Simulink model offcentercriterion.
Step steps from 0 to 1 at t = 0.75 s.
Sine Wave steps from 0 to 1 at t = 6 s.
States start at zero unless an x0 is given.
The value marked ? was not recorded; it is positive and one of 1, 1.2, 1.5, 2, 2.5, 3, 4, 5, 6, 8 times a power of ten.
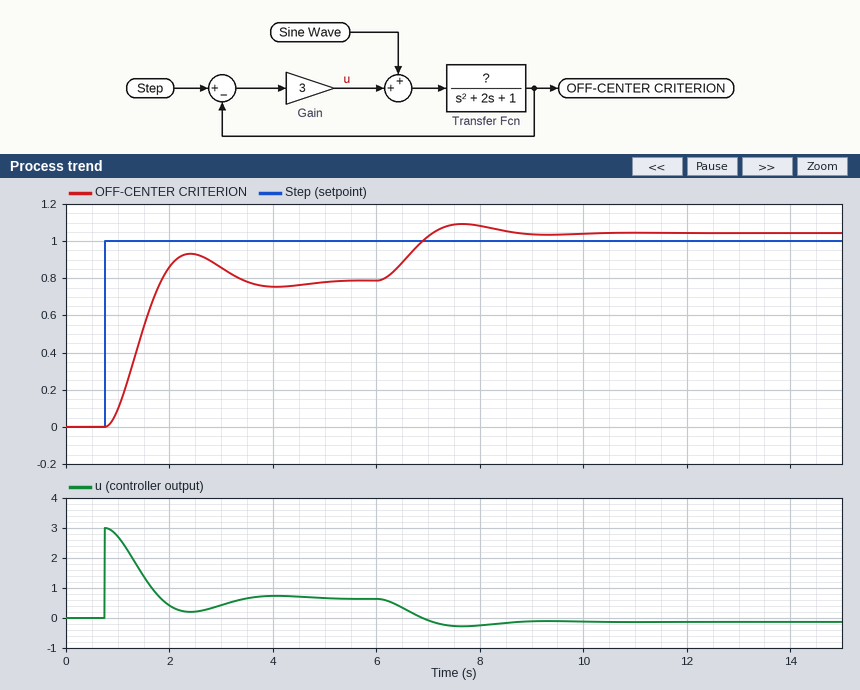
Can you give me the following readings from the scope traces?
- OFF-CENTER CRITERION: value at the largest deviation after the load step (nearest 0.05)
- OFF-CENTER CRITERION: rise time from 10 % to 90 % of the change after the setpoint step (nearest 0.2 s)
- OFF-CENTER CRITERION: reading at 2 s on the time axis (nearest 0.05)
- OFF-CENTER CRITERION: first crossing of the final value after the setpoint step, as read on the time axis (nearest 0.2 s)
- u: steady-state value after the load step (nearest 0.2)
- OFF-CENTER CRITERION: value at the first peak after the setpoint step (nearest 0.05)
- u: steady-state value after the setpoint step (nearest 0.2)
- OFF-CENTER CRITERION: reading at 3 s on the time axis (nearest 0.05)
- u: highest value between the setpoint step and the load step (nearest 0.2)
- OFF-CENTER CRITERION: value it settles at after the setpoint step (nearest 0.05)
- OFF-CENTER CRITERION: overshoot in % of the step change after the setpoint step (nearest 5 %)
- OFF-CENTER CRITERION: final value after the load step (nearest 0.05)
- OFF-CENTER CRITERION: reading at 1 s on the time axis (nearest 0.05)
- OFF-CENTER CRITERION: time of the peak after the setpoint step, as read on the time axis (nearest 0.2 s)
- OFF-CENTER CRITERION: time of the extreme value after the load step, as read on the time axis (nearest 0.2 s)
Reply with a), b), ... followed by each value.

a) 1.10
b) 0.8 s
c) 0.85
d) 1.8 s
e) -0.2
f) 0.95
g) 0.6
h) 0.85
i) 3.0
j) 0.80
k) 20 %
l) 1.05
m) 0.10
n) 2.4 s
o) 7.6 s
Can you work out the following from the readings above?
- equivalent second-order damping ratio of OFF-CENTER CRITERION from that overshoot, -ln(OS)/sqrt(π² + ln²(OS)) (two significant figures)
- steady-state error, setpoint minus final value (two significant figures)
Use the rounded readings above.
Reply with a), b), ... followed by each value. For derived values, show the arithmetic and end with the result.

a) ln(0.2) = -1.609; 1.609 / sqrt(9.870 + 2.590) = 0.46
b) 1 - 0.8 = 0.20
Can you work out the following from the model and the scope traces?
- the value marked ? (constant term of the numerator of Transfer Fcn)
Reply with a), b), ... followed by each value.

a) 1.2
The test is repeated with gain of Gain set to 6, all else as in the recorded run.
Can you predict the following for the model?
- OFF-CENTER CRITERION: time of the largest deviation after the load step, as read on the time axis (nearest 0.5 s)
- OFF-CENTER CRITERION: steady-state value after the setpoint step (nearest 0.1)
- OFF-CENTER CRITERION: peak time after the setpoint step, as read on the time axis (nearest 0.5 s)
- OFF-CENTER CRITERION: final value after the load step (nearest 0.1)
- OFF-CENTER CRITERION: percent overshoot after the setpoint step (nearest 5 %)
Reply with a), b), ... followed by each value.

a) 7.0 s
b) 0.9
c) 2.0 s
d) 1.0
e) 30 %
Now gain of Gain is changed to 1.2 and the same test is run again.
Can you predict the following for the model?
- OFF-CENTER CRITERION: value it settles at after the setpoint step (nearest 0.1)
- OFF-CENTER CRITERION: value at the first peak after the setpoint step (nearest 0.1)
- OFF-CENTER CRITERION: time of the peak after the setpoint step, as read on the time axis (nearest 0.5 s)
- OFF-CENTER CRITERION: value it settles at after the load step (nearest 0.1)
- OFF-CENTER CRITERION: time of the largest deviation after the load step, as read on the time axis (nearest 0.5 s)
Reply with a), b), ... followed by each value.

a) 0.6
b) 0.6
c) 3.5 s
d) 1.1
e) 8.5 s
